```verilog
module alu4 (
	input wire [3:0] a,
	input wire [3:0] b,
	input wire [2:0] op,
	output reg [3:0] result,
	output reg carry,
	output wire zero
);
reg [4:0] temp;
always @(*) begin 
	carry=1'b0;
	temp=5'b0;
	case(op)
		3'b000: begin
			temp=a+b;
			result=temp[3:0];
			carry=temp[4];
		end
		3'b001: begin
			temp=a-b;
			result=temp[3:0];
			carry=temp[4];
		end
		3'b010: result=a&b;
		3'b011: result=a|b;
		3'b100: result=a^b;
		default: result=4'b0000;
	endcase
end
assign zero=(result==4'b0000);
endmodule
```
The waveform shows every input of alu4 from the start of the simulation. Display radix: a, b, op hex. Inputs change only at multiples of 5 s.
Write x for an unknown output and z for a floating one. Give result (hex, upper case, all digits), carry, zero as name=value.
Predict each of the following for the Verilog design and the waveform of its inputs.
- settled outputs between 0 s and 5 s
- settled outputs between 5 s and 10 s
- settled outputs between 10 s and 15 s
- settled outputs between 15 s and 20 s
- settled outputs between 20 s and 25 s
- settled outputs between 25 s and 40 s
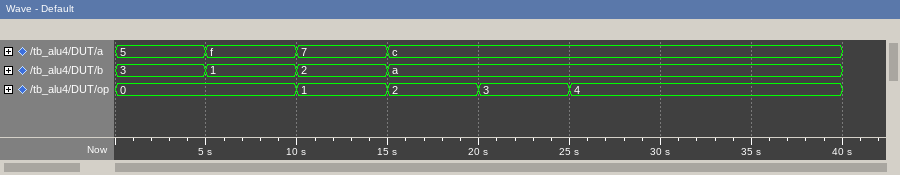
result=8, carry=0, zero=0
result=0, carry=1, zero=1
result=5, carry=0, zero=0
result=8, carry=0, zero=0
result=E, carry=0, zero=0
result=6, carry=0, zero=0
